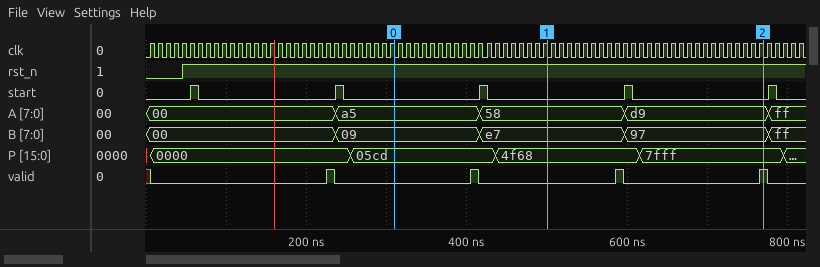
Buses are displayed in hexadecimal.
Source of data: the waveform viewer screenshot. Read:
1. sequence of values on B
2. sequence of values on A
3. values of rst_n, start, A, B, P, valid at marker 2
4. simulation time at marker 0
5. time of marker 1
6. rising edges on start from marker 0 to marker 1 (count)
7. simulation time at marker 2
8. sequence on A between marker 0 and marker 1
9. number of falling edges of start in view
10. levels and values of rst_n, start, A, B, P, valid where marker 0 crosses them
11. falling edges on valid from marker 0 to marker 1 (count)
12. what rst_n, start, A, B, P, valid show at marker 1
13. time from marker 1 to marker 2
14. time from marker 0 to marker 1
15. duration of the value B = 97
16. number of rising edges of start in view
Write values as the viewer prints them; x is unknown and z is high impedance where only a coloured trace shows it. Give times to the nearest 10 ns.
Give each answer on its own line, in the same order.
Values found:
00, 09, e7, 97, ff
00, a5, 58, d9, ff
rst_n=1, start=0, A=d9, B=97, P=7fff, valid=1
310 ns
500 ns
1
770 ns
a5, 58
5
rst_n=1, start=0, A=a5, B=09, P=05cd, valid=0
1
rst_n=1, start=0, A=58, B=e7, P=4f68, valid=0
270 ns
190 ns
180 ns
5
